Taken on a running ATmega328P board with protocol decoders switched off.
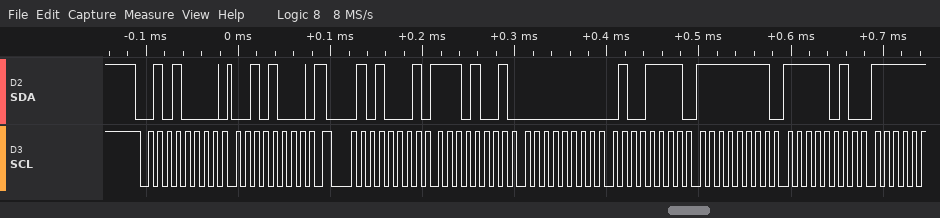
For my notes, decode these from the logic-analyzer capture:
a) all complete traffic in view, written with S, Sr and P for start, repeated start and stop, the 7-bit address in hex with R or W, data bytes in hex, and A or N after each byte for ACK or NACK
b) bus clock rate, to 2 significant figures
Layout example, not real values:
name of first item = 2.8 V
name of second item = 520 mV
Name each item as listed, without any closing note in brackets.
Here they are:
all complete traffic in view, written with S, Sr and P for start, repeated start and stop, the 7-bit address in hex with R or W, data bytes in hex, and A or N after each byte for ACK or NACK = S 28W A 28 A Sr 28R A E9 A 00 A 4F A FF A FA A
bus clock rate, to 2 significant figures = 100 kHz
